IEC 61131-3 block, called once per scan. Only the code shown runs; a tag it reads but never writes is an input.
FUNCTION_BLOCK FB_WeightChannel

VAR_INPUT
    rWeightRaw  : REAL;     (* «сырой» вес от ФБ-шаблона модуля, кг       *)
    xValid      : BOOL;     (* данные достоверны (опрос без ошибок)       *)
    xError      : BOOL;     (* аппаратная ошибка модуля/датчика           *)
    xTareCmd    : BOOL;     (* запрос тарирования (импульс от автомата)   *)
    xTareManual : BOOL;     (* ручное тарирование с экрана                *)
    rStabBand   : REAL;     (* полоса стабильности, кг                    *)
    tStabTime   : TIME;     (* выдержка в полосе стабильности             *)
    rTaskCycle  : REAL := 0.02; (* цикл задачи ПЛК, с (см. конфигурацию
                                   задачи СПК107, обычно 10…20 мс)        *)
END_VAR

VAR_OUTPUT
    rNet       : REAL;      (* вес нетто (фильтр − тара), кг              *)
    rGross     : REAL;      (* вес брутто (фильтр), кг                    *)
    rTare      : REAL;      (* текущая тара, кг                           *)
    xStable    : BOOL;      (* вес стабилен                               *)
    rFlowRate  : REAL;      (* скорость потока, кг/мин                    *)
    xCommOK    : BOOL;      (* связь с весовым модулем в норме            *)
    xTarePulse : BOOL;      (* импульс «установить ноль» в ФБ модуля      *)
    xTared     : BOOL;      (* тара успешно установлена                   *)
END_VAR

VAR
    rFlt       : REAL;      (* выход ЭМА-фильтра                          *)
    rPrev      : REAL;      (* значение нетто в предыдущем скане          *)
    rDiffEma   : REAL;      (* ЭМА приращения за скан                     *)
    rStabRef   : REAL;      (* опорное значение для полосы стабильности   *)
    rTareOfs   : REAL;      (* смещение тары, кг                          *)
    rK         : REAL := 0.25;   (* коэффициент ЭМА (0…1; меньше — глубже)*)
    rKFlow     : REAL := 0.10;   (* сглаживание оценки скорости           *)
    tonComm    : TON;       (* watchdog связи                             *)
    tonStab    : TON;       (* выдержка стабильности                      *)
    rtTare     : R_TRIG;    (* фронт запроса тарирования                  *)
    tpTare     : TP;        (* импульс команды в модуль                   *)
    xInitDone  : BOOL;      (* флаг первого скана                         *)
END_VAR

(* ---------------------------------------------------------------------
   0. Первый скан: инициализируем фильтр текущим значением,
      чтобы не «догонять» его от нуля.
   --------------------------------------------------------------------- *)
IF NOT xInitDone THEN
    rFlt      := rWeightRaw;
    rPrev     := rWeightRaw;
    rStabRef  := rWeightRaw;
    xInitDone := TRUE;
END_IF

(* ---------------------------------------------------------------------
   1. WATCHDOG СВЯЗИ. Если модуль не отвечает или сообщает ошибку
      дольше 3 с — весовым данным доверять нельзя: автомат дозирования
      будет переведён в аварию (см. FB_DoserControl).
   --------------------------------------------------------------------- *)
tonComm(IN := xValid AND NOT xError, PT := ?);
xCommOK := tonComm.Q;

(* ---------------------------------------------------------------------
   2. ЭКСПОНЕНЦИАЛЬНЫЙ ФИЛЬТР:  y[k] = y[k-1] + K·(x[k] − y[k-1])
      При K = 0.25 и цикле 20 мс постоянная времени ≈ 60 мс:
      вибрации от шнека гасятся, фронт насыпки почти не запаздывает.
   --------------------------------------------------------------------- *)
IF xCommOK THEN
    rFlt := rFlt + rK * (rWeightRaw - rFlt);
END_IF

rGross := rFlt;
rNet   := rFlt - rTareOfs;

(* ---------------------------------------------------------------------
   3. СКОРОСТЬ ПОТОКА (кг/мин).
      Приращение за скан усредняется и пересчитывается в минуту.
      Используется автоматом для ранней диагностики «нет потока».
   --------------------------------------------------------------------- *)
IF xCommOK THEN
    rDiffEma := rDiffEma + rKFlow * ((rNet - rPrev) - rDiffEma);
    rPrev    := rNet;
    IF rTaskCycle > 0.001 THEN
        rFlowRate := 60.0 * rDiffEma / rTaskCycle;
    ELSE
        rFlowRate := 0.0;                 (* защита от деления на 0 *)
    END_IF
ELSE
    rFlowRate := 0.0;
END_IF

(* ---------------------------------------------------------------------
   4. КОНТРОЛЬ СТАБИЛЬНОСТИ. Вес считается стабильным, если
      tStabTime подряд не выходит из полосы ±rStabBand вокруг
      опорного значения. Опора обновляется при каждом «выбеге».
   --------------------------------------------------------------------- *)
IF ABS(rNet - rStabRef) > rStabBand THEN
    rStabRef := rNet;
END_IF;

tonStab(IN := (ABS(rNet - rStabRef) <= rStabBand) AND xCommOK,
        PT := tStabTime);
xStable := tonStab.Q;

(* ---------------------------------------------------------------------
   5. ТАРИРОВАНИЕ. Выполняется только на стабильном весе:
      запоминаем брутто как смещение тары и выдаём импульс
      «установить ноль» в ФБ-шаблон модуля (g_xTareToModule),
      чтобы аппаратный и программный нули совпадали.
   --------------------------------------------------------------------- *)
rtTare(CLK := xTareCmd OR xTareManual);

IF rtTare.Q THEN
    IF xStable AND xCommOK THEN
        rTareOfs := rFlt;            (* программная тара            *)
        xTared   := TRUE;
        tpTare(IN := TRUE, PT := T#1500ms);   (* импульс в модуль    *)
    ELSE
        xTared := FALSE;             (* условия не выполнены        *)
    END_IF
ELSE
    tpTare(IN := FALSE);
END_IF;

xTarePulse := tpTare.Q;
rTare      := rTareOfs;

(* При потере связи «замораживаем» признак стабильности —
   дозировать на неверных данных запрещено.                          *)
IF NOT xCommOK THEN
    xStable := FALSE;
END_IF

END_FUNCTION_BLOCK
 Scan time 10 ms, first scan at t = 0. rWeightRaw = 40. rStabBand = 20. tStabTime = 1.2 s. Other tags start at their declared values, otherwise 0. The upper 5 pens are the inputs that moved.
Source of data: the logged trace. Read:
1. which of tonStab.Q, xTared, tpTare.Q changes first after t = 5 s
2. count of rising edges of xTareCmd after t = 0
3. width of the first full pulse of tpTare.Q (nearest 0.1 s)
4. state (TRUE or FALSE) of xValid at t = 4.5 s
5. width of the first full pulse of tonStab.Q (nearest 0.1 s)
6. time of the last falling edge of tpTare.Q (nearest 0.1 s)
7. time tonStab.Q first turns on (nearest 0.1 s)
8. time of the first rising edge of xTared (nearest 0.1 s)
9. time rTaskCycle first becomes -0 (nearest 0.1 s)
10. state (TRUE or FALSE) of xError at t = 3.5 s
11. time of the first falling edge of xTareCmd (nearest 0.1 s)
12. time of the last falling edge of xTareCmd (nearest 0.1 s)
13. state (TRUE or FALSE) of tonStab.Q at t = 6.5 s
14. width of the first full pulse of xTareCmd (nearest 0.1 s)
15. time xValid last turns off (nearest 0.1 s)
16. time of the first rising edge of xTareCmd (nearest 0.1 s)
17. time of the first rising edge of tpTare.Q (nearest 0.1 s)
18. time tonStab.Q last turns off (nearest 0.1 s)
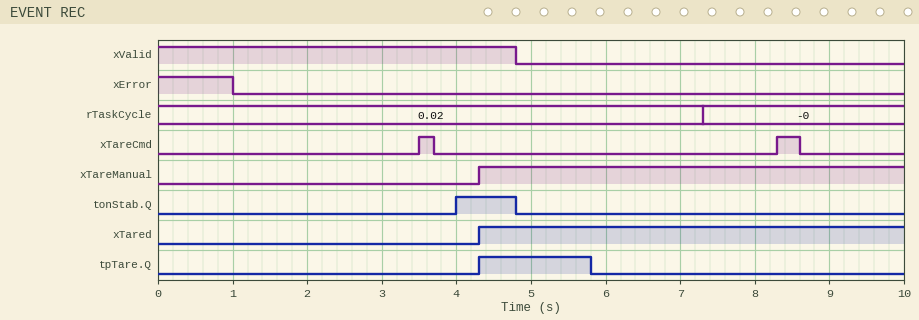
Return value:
tpTare.Q
2
1.5 s
TRUE
0.8 s
5.8 s
4.0 s
4.3 s
7.3 s
FALSE
3.7 s
8.6 s
FALSE
0.2 s
4.8 s
3.5 s
4.3 s
4.8 s
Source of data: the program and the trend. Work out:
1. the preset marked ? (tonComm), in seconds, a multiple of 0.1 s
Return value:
1.8 s
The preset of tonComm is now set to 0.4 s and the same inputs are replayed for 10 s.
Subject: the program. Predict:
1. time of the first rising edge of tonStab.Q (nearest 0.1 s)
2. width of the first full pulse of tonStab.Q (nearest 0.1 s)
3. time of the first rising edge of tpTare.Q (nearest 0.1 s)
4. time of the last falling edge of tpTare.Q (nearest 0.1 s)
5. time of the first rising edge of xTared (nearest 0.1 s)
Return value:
2.6 s
2.2 s
3.5 s
5.0 s
3.5 s
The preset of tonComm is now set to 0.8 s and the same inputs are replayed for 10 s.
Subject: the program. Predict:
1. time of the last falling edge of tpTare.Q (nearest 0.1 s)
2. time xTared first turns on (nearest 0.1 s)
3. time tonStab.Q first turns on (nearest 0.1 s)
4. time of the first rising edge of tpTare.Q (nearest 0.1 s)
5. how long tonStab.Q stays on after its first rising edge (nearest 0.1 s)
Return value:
5.0 s
3.5 s
3.0 s
3.5 s
1.8 s
